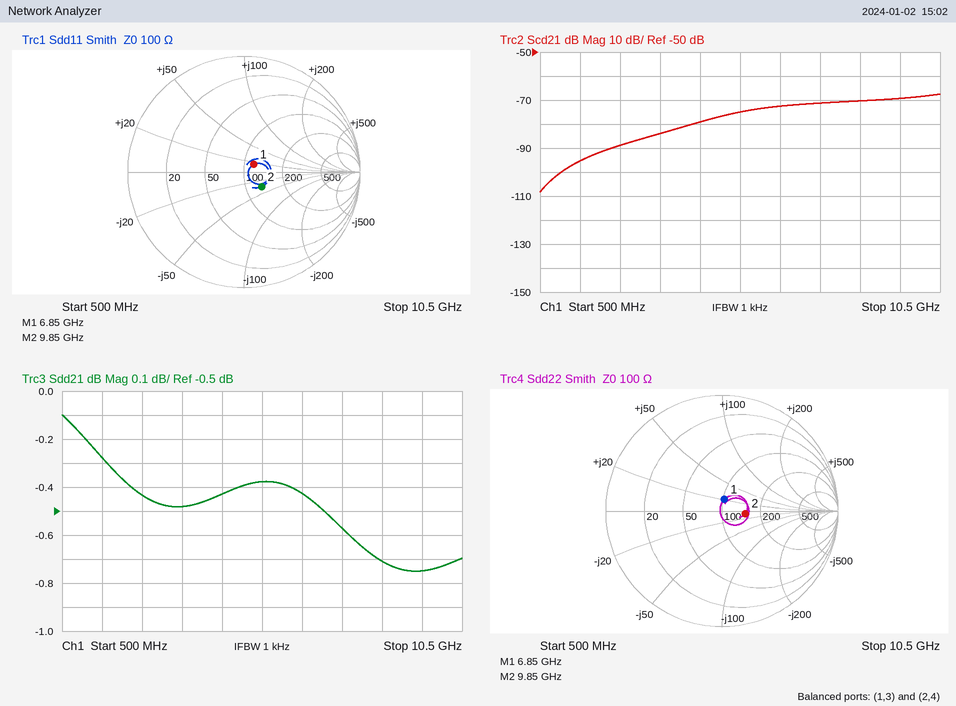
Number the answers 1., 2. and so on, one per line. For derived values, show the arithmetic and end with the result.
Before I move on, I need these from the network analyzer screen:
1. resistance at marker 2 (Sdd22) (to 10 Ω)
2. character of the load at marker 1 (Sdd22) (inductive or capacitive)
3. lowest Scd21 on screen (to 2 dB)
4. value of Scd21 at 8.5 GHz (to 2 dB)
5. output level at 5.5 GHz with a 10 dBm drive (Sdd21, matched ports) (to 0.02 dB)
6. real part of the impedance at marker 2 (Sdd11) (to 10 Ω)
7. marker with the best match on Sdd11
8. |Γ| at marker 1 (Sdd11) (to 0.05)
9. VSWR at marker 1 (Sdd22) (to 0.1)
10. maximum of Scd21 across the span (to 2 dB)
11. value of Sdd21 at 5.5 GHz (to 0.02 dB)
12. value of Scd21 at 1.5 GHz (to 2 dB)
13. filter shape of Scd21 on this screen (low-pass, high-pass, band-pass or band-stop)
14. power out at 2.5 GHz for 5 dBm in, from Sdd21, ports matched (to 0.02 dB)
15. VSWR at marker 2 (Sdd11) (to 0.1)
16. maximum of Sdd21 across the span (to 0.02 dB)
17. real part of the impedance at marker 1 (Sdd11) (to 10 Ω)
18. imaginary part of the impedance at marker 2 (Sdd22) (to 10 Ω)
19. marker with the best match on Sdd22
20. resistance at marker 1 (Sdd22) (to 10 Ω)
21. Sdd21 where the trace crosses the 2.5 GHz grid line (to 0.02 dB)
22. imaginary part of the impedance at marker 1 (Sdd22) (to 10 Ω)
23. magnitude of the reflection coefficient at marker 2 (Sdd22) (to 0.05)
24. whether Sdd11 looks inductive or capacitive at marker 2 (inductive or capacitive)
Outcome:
1. 150 Ω
2. inductive
3. -108 dB
4. -70 dB
5. 10 dBm + (-0.38 dB) = 9.62 dBm
6. 130 Ω
7. marker 1
8. 0.10
9. 1.2
10. -68 dB
11. -0.38 dB
12. -96 dB
13. high-pass
14. 5 dBm + (-0.44 dB) = 4.56 dBm
15. 1.5
16. -0.10 dB
17. 120 Ω
18. -10 Ω
19. marker 1
20. 100 Ω
21. -0.44 dB
22. +20 Ω
23. 0.20
24. capacitive
